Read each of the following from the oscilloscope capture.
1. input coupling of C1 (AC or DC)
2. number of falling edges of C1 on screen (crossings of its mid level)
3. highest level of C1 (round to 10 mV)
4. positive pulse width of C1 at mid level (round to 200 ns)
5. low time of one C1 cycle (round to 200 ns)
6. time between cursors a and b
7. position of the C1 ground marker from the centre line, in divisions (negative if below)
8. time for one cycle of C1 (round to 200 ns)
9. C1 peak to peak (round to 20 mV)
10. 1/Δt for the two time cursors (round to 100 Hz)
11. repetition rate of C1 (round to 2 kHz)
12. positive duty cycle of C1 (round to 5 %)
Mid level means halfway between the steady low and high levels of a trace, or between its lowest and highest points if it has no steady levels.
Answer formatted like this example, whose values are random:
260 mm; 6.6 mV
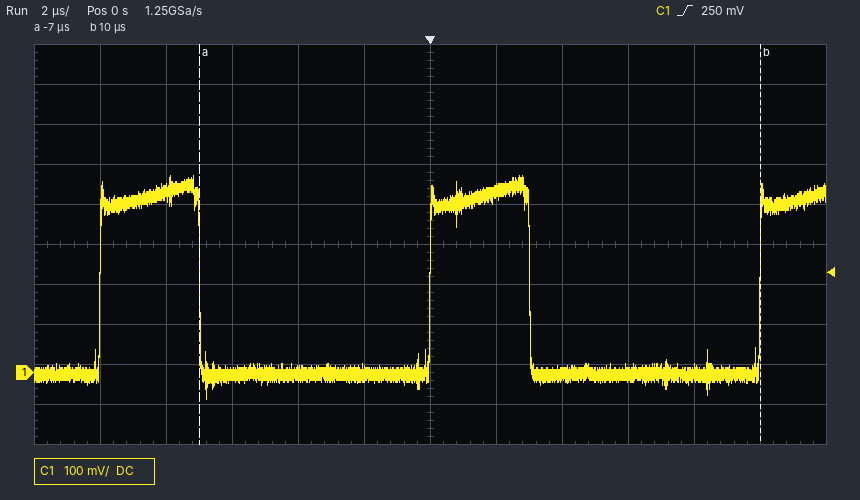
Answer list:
DC; 2; 490 mV; 3.0 µs; 7.0 µs; 17.0 µs; -3.2 div; 10.0 µs; 560 mV; 58.8 kHz; 100 kHz; 30 %
